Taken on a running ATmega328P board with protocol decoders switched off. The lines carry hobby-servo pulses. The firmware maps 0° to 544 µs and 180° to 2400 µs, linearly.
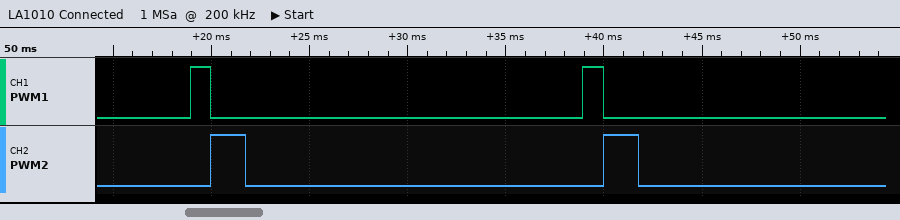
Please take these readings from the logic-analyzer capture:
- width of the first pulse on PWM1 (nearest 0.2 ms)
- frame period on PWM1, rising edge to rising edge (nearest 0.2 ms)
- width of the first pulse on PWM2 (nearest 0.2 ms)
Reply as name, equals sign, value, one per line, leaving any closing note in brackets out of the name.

width of the first pulse on PWM1 = 1.0 ms
frame period on PWM1, rising edge to rising edge = 20.0 ms
width of the first pulse on PWM2 = 1.8 ms
